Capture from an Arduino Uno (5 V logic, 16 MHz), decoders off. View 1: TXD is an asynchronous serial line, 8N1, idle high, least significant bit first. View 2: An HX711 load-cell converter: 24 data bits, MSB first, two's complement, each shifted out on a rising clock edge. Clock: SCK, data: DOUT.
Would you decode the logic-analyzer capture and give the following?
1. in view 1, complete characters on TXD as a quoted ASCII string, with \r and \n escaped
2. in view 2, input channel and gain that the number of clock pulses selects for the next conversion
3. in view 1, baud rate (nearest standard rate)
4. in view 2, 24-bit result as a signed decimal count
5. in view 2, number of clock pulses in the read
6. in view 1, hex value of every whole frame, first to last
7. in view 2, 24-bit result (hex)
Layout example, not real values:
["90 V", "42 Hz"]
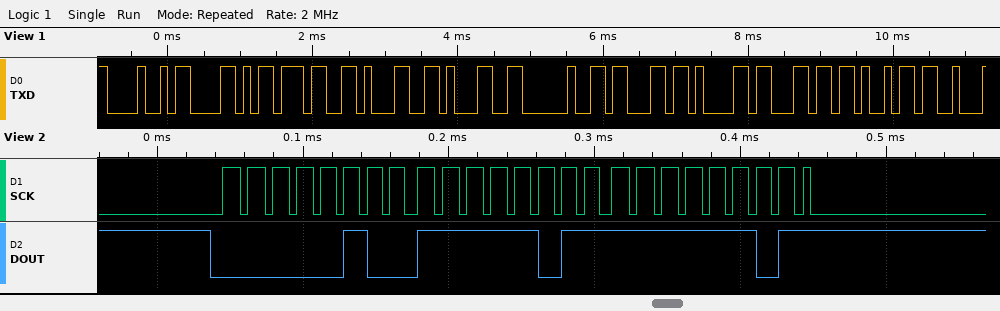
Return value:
["\"HX711 cali\"", "channel A, gain 128", "9600 baud", "326653", "25", "48 58 37 31 31 20 63 61 6C 69", "0x04FBFD"]
